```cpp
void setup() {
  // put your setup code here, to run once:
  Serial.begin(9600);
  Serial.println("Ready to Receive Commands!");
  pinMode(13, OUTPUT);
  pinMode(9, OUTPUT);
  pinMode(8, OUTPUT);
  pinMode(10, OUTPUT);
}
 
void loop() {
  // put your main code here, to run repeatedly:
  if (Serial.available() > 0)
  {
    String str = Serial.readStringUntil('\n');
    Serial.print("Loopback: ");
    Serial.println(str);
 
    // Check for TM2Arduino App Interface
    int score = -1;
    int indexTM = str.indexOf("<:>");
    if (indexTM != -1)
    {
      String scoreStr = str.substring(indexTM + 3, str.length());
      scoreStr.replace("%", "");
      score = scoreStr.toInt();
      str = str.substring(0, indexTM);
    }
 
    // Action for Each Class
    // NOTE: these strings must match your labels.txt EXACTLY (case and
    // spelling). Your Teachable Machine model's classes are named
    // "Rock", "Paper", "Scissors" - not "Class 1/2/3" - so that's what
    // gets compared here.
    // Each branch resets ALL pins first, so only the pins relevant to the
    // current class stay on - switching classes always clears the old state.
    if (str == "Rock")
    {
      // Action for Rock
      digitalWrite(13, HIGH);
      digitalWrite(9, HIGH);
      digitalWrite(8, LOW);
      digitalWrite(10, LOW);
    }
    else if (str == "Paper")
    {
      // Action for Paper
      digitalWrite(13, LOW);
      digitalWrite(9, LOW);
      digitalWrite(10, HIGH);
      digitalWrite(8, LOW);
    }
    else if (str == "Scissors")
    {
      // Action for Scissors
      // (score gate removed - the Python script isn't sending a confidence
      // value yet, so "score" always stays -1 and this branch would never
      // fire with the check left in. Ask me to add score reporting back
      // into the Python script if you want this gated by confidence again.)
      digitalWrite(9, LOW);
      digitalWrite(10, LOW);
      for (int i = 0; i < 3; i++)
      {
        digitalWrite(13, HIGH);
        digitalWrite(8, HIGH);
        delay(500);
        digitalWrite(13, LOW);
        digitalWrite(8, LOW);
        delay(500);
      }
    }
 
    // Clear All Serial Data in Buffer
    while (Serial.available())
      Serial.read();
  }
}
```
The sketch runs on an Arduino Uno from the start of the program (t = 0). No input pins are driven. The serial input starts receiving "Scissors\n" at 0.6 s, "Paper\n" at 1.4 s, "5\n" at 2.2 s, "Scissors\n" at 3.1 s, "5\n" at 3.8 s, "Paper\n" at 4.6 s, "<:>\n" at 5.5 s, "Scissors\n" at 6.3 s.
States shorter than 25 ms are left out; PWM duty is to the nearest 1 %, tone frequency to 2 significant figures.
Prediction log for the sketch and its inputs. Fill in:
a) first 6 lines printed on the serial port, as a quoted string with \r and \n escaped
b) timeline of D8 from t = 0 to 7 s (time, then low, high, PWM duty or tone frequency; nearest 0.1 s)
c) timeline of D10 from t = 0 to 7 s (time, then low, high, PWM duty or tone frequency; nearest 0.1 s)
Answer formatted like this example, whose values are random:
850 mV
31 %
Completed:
"Ready to Receive Commands!\r\nLoopback: Scissors\r\nLoopback: 5\r\nLoopback: Paper\r\nLoopback: <:>\r\nLoopback: Scissors\r\n"
0 s low; 0.6 s high; 1.1 s low; 1.6 s high; 2.1 s low; 2.6 s high; 3.1 s low; 6.3 s high; 6.8 s low
0 s low; 4.6 s high; 6.3 s low
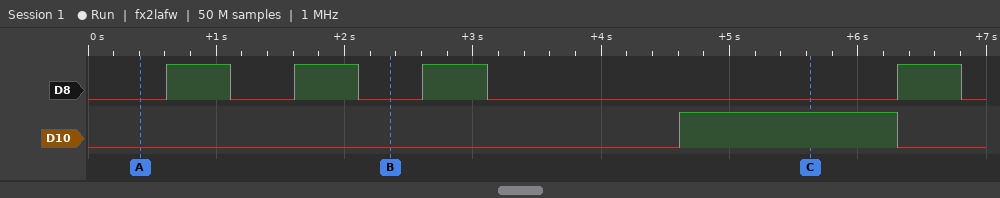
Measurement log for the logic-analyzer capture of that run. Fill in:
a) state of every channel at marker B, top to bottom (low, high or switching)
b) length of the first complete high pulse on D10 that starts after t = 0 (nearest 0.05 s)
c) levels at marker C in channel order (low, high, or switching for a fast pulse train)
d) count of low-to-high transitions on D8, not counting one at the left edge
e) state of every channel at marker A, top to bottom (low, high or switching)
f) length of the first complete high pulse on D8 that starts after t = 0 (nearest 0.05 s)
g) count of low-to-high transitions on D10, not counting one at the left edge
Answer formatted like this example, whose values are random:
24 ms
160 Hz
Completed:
D8 low, D10 low
1.70 s
D8 low, D10 high
4
D8 low, D10 low
0.50 s
1
